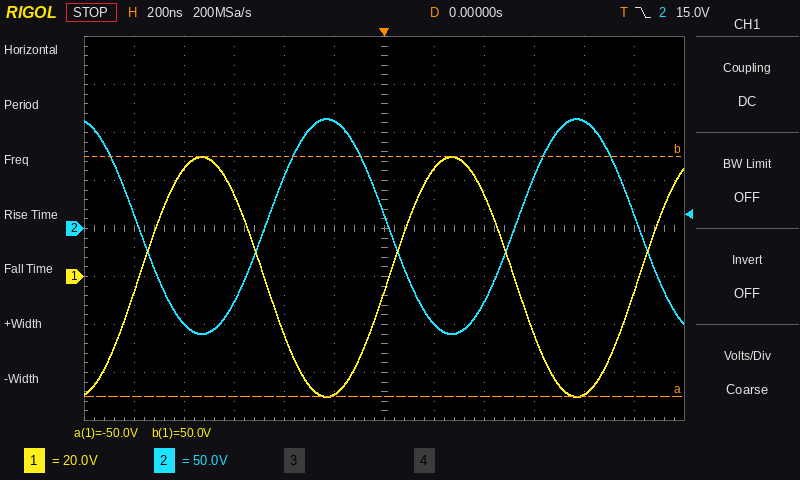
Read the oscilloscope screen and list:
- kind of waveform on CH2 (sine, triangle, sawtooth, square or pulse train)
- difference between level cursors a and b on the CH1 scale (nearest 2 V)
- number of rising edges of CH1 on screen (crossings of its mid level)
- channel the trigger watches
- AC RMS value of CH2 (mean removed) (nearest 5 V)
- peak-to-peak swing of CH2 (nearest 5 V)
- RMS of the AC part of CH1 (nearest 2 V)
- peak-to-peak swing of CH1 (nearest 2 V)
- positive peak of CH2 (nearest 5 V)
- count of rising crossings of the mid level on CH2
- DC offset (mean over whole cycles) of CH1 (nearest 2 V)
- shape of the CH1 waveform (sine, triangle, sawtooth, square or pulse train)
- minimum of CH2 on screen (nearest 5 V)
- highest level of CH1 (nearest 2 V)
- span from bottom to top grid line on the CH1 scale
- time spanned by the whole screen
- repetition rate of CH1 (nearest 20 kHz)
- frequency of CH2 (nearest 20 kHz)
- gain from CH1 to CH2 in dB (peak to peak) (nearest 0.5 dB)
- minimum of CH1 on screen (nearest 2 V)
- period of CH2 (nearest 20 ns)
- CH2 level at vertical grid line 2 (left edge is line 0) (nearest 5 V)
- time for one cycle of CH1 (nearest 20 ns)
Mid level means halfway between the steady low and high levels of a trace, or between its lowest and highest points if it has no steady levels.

sine
100 V
3
CH2
80 V
225 V
36 V
100 V
115 V
2
0 V
sine
-110 V
50 V
160 V
2.4 µs
1.00 MHz
1.00 MHz
7.0 dB
-50 V
1.00 µs
-100 V
1.00 µs
